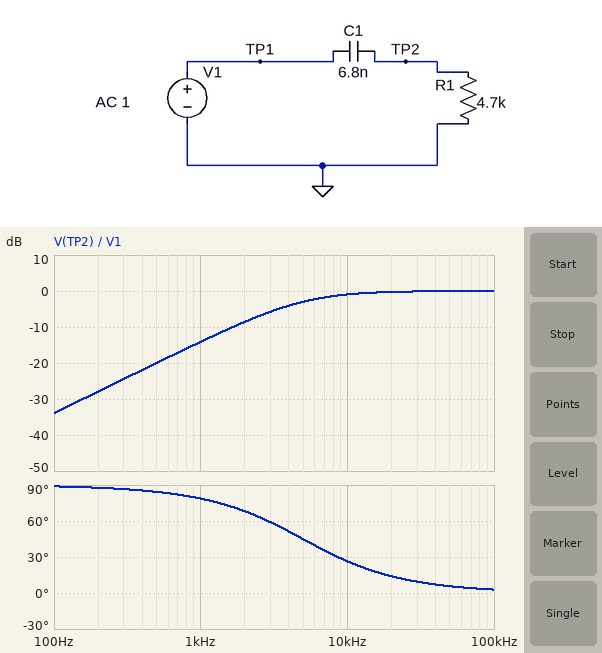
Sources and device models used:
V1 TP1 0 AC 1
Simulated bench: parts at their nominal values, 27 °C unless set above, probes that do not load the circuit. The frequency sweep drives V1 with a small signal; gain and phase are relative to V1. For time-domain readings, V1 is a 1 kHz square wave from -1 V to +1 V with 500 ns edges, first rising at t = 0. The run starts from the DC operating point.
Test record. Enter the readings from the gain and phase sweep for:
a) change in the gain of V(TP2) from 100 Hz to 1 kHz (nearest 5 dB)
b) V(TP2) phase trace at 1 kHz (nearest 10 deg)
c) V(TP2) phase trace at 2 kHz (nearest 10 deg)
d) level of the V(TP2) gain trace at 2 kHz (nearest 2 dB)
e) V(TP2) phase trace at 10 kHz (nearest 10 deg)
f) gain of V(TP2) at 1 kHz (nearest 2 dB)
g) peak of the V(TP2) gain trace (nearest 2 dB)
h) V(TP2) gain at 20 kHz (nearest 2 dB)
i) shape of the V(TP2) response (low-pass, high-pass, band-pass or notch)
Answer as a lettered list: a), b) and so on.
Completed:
a) 20 dB
b) 80 deg
c) 70 deg
d) -8 dB
e) 30 deg
f) -14 dB
g) 0 dB
h) 0 dB
i) high-pass
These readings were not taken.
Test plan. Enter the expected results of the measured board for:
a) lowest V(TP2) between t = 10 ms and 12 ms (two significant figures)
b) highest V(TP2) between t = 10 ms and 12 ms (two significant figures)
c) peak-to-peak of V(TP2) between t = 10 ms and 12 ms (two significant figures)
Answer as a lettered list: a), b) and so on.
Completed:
a) -2.0 V
b) 2.0 V
c) 4.0 V
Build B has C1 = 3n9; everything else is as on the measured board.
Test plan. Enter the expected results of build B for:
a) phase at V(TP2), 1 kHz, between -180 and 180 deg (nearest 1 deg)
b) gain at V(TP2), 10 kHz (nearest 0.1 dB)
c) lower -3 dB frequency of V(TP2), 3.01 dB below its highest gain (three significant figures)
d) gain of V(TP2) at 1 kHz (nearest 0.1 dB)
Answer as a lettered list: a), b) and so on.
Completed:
a) 83 deg
b) -2.4 dB
c) 8.68 kHz
d) -18.8 dB
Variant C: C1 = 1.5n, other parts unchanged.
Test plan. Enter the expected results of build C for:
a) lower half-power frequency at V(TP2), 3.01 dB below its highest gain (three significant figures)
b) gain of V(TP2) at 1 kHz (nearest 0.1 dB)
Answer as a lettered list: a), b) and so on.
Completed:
a) 22.6 kHz
b) -27.1 dB
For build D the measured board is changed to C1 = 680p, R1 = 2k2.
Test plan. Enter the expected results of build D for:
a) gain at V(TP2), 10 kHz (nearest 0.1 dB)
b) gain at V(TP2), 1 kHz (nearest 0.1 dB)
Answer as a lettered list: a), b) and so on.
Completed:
a) -20.6 dB
b) -40.5 dB
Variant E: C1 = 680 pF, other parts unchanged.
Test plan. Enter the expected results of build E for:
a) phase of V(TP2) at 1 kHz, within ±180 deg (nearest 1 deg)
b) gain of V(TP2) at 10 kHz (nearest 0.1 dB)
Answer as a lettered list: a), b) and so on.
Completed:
a) 89 deg
b) -14.1 dB
